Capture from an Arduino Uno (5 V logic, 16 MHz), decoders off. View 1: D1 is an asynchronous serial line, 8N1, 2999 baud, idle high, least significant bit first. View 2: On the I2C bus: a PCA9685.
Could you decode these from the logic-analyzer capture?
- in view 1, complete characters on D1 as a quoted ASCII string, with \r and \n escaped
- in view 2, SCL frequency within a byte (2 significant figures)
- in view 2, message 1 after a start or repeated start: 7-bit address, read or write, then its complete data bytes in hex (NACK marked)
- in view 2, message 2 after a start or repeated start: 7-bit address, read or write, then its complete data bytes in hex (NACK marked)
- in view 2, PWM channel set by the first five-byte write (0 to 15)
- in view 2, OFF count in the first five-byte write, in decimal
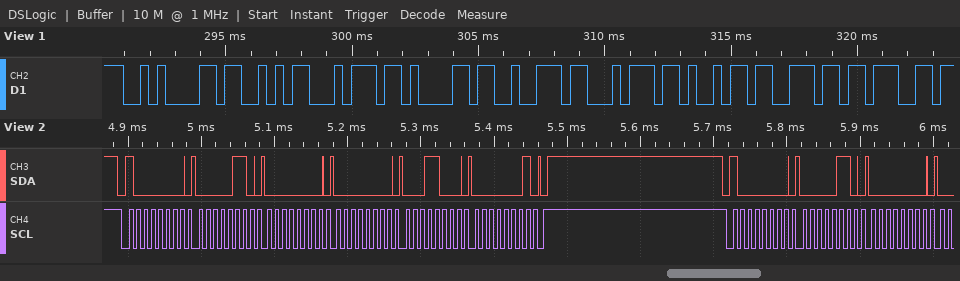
"\nStarting"
100 kHz
0x40 write: 06 00 00 18 01
0x40 write: 06 00
0
280
